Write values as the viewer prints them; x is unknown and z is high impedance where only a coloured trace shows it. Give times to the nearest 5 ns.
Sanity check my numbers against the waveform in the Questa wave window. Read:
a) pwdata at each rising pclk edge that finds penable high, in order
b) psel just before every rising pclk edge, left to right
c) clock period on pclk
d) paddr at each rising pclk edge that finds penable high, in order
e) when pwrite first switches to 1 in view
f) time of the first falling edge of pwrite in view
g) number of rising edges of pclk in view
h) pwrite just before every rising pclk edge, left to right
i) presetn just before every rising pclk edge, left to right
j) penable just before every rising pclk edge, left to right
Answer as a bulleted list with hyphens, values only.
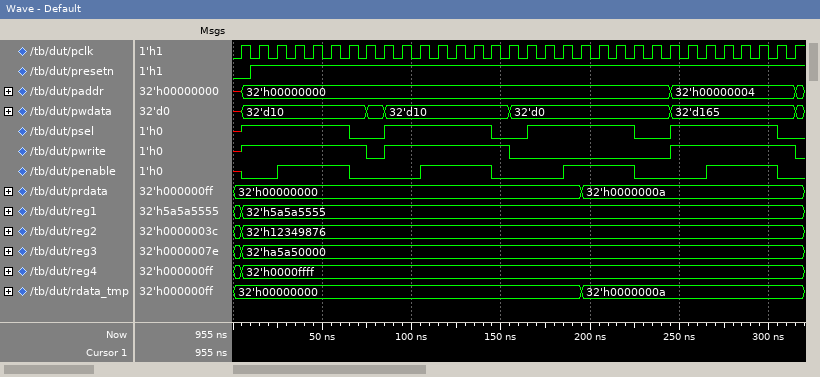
- 32'd10, 32'd10, 32'd10, 32'd10, 32'd10, 32'd10, 32'd10, 32'd10, 32'd0, 32'd0, 32'd0, 32'd0, 32'd165, 32'd165, 32'd165, 32'd165
- x 1 1 1 1 1 1 0 0 1 1 1 1 1 1 0 0 1 1 1 1 1 1 0 0 1 1 1 1 1 1 0
- 10 ns
- 32'h00000000, 32'h00000000, 32'h00000000, 32'h00000000, 32'h00000000, 32'h00000000, 32'h00000000, 32'h00000000, 32'h00000000, 32'h00000000, 32'h00000000, 32'h00000000, 32'h00000004, 32'h00000004, 32'h00000004, 32'h00000004
- 5 ns
- 75 ns
- 32
- x 1 1 1 1 1 1 1 0 1 1 1 1 1 1 1 0 0 0 0 0 0 0 0 0 1 1 1 1 1 1 1
- 0 1 1 1 1 1 1 1 1 1 1 1 1 1 1 1 1 1 1 1 1 1 1 1 1 1 1 1 1 1 1 1
- x 0 0 1 1 1 1 0 0 0 0 1 1 1 1 0 0 0 0 1 1 1 1 0 0 0 0 1 1 1 1 0
